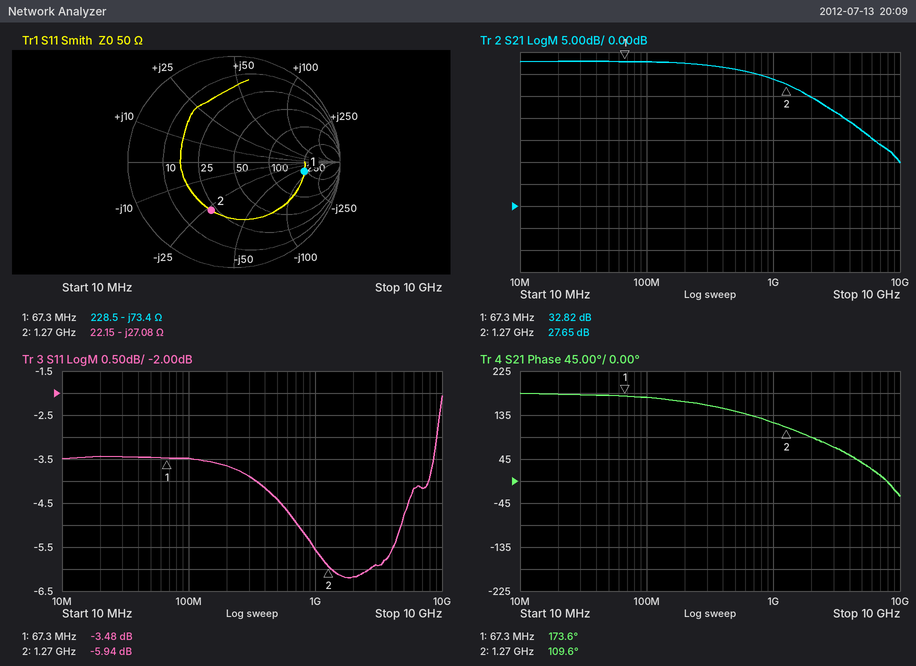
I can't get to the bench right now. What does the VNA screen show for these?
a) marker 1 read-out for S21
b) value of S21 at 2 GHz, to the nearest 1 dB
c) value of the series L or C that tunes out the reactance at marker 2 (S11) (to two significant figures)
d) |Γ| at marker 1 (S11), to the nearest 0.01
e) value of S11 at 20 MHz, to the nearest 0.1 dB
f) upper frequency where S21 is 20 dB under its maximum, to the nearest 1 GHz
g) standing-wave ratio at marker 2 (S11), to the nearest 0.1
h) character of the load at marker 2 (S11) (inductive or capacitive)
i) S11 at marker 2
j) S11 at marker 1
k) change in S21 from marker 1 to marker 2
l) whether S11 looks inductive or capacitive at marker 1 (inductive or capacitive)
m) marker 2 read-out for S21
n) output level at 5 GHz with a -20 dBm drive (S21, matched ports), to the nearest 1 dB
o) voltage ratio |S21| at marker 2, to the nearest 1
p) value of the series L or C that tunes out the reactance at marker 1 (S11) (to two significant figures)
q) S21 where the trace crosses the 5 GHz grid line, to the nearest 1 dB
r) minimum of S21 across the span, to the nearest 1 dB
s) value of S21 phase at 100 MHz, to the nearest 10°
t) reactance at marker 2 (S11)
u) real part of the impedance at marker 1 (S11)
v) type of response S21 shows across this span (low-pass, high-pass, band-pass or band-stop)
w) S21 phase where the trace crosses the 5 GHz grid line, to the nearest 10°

32.82 dB
25 dB
3.4 nH
0.67
-3.4 dB
8 GHz
3.0
capacitive
-5.94 dB
-3.48 dB
-5.17 dB
capacitive
27.65 dB
-3 dBm
24
170 nH
17 dB
10 dB
170°
-27.08 Ω
228.5 Ω
low-pass
40°
